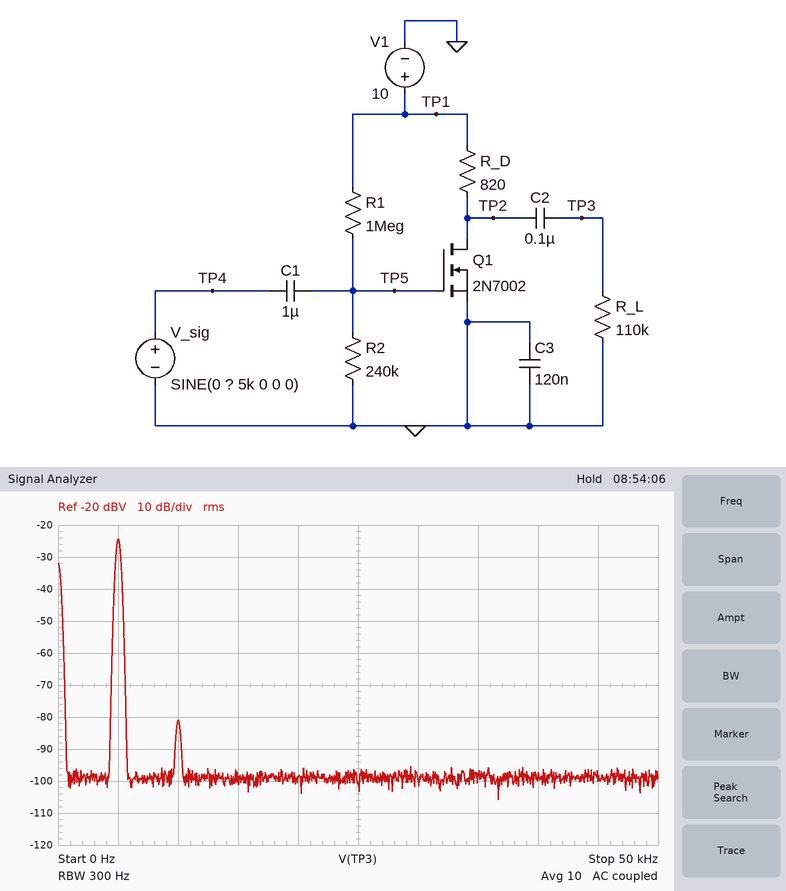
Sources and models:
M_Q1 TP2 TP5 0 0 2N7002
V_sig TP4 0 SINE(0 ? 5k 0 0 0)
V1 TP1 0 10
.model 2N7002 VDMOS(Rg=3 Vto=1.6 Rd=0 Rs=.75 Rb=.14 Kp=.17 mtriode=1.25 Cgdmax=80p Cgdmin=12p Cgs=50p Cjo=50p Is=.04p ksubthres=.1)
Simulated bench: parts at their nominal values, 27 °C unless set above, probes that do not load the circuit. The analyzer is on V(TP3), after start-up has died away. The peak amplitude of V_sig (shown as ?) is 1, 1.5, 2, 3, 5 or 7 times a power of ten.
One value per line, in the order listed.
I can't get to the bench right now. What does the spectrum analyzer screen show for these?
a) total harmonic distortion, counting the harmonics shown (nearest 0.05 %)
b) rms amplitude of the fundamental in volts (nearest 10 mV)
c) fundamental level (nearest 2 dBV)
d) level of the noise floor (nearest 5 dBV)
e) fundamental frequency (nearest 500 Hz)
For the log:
0.15 %
60 mV
-24 dBV
-100 dBV
5.0 kHz
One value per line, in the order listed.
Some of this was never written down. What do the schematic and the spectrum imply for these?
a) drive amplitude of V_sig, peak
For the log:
2 mV
